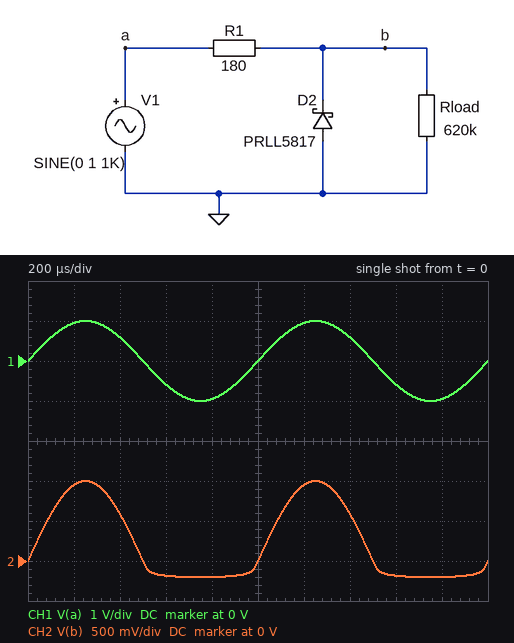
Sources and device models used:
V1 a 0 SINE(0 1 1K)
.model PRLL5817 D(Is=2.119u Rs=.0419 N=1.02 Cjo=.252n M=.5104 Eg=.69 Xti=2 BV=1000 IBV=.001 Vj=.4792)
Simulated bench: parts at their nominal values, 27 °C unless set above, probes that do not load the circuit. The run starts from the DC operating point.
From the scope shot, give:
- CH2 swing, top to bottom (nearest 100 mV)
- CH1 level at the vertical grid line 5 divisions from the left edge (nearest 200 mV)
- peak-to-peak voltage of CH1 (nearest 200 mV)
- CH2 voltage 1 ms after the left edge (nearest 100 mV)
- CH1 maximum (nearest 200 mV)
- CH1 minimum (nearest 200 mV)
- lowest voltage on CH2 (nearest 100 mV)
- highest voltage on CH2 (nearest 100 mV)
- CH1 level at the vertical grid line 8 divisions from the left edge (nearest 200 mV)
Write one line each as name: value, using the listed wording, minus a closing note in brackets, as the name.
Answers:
CH2 swing, top to bottom: 1.2 V
CH1 level at the vertical grid line 5 divisions from the left edge: 0 V
peak-to-peak voltage of CH1: 2.0 V
CH2 voltage 1 ms after the left edge: 0 V
CH1 maximum: 1.0 V
CH1 minimum: -1.0 V
lowest voltage on CH2: -200 mV
highest voltage on CH2: 1.0 V
CH1 level at the vertical grid line 8 divisions from the left edge: -600 mV
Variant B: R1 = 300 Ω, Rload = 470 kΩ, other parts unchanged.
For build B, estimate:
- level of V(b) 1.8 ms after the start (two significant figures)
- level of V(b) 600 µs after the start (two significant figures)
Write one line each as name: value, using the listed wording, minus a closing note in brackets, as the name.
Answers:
level of V(b) 1.8 ms after the start: -190 mV
level of V(b) 600 µs after the start: -170 mV
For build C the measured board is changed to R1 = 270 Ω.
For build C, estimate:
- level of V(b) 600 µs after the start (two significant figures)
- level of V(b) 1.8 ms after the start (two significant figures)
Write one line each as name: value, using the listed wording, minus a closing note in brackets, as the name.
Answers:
level of V(b) 600 µs after the start: -170 mV
level of V(b) 1.8 ms after the start: -190 mV
